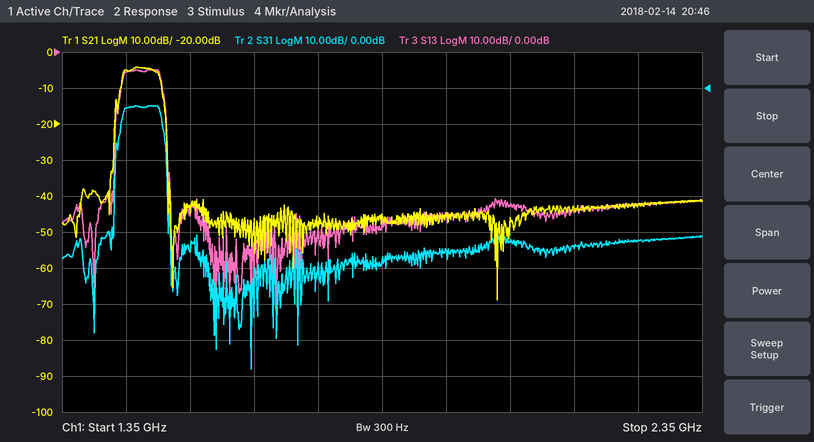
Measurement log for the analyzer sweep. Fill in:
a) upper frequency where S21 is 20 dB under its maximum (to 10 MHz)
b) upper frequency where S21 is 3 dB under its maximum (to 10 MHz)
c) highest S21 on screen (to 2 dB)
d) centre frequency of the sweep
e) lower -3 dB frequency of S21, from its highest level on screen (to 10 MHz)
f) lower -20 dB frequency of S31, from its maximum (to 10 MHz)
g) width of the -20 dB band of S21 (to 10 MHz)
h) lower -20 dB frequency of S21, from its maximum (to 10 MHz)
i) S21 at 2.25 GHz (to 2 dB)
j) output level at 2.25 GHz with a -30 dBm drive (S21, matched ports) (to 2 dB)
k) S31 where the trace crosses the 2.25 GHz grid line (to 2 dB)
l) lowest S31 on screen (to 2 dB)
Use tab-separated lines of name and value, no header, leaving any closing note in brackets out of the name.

upper frequency where S21 is 20 dB under its maximum	1.51 GHz
upper frequency where S21 is 3 dB under its maximum	1.50 GHz
highest S21 on screen	-4 dB
centre frequency of the sweep	1.85 GHz
lower -3 dB frequency of S21, from its highest level on screen	1.44 GHz
lower -20 dB frequency of S31, from its maximum	1.43 GHz
width of the -20 dB band of S21	80 MHz
lower -20 dB frequency of S21, from its maximum	1.43 GHz
S21 at 2.25 GHz	-42 dB
output level at 2.25 GHz with a -30 dBm drive (S21, matched ports)	-72 dBm
S31 where the trace crosses the 2.25 GHz grid line	-42 dB
lowest S31 on screen	-78 dB
